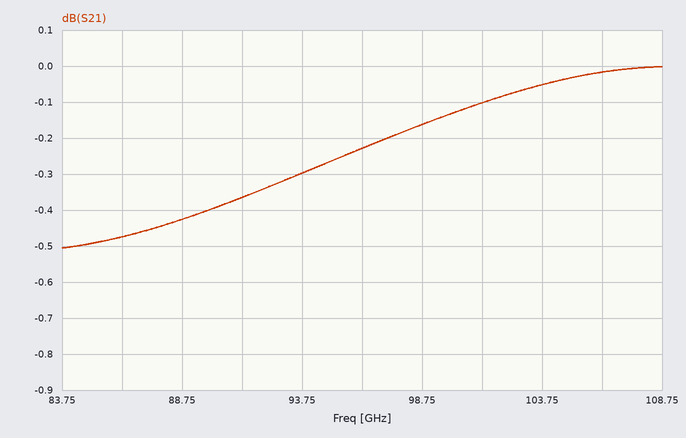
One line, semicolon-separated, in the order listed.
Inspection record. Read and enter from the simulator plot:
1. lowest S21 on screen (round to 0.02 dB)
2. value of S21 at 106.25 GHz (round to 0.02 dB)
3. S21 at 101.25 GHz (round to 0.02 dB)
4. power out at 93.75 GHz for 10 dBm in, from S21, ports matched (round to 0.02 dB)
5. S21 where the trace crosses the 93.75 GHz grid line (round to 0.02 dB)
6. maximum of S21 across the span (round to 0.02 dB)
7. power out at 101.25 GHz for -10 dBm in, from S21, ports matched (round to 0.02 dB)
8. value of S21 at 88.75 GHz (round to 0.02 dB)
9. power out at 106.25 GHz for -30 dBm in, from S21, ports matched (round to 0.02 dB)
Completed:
-0.50 dB; -0.02 dB; -0.10 dB; 9.70 dBm; -0.30 dB; 0.00 dB; -10.10 dBm; -0.42 dB; -30.02 dBm
